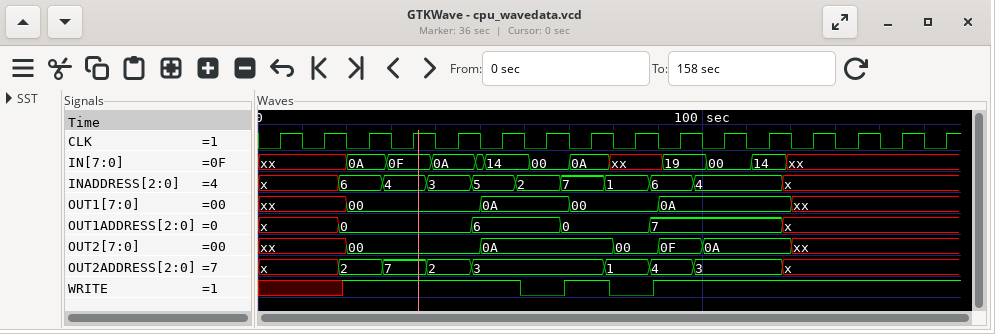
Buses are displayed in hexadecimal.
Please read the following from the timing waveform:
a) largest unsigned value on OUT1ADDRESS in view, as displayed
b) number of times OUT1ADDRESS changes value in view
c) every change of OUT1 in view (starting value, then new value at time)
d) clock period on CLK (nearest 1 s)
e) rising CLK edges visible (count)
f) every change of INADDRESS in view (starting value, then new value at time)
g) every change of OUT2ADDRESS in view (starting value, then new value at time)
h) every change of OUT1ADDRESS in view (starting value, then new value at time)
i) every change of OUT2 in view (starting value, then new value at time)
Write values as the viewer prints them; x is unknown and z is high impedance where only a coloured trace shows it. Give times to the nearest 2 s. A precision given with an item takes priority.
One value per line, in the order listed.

7
5
xx, 00 at 20 s, 0A at 50 s, 00 at 70 s, 0A at 90 s, xx at 120 s
10 s
16
x, 6 at 18 s, 4 at 28 s, 3 at 38 s, 5 at 48 s, 2 at 58 s, 7 at 68 s, 1 at 78 s, 6 at 88 s, 4 at 98 s, x at 118 s
x, 2 at 18 s, 7 at 28 s, 2 at 38 s, 3 at 48 s, 1 at 78 s, 4 at 88 s, 3 at 98 s, x at 118 s
x, 0 at 18 s, 6 at 48 s, 0 at 68 s, 7 at 88 s, x at 118 s
xx, 00 at 20 s, 0A at 50 s, 00 at 80 s, 0F at 90 s, 0A at 100 s, xx at 120 s
